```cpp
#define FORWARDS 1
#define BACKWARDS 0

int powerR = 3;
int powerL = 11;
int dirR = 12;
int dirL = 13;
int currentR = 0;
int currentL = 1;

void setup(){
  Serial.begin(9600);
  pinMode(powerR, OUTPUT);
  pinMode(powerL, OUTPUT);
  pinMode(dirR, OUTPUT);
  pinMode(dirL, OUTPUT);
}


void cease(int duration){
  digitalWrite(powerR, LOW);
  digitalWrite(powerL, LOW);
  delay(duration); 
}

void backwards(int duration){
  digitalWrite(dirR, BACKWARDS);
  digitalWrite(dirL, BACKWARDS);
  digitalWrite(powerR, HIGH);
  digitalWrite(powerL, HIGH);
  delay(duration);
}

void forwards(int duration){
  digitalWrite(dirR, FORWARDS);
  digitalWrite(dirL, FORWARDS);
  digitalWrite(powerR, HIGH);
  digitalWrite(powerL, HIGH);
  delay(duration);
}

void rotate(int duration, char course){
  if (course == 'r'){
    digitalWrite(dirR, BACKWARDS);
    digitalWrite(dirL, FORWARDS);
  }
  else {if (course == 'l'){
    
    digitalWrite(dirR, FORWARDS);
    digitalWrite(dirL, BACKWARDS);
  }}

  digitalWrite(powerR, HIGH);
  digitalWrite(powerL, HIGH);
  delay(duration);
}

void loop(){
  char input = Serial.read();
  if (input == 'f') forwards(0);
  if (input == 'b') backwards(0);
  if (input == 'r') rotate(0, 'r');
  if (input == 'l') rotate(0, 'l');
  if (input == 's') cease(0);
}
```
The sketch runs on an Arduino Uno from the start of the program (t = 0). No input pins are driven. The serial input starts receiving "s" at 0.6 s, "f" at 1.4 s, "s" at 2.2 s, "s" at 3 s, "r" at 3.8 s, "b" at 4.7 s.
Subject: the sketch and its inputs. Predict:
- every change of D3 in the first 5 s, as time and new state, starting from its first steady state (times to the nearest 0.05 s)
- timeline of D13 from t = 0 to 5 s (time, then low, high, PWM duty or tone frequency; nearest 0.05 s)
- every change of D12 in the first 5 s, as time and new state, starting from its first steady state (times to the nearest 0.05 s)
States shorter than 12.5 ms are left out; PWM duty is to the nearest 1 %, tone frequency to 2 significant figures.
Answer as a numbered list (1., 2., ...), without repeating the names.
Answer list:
1. 0 s low; 1.4 s high; 2.2 s low; 3.8 s high
2. 0 s low; 1.4 s high; 4.7 s low
3. 0 s low; 1.4 s high; 3.8 s low
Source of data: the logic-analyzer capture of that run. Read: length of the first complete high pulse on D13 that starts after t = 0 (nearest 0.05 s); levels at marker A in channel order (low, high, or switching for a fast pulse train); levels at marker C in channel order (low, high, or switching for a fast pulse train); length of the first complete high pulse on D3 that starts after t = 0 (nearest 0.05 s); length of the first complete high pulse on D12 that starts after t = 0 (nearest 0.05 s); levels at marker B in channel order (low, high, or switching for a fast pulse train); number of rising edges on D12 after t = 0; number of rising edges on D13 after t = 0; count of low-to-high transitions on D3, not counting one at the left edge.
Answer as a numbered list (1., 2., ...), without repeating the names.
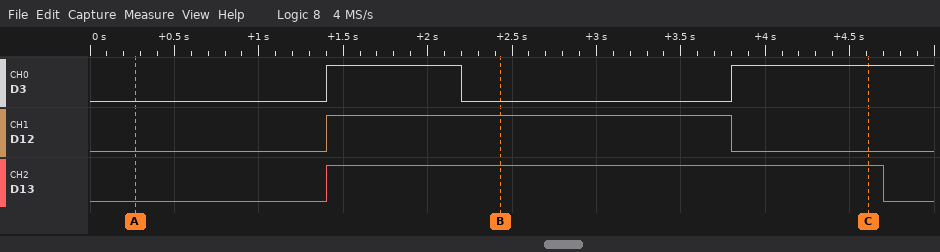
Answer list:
1. 3.30 s
2. D3 low, D12 low, D13 low
3. D3 high, D12 low, D13 high
4. 0.80 s
5. 2.40 s
6. D3 low, D12 high, D13 high
7. 1
8. 1
9. 2
